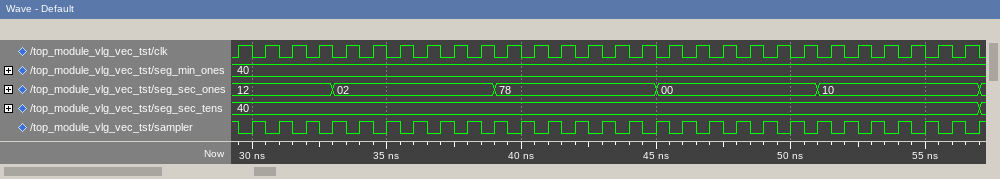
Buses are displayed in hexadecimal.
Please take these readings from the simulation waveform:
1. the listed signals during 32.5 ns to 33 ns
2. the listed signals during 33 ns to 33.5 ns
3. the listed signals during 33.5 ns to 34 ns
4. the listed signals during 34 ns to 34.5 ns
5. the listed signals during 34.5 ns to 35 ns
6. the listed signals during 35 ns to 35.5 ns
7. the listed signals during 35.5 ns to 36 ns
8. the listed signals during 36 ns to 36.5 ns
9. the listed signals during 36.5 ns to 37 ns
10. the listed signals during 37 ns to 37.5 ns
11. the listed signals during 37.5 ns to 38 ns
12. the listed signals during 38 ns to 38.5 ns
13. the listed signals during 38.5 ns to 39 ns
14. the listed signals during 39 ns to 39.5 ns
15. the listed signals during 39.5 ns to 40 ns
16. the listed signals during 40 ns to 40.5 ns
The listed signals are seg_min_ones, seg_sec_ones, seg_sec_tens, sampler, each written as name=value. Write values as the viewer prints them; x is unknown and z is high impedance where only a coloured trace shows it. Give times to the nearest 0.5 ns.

seg_min_ones=40, seg_sec_ones=12, seg_sec_tens=40, sampler=0
seg_min_ones=40, seg_sec_ones=02, seg_sec_tens=40, sampler=1
seg_min_ones=40, seg_sec_ones=02, seg_sec_tens=40, sampler=0
seg_min_ones=40, seg_sec_ones=02, seg_sec_tens=40, sampler=1
seg_min_ones=40, seg_sec_ones=02, seg_sec_tens=40, sampler=0
seg_min_ones=40, seg_sec_ones=02, seg_sec_tens=40, sampler=1
seg_min_ones=40, seg_sec_ones=02, seg_sec_tens=40, sampler=0
seg_min_ones=40, seg_sec_ones=02, seg_sec_tens=40, sampler=1
seg_min_ones=40, seg_sec_ones=02, seg_sec_tens=40, sampler=0
seg_min_ones=40, seg_sec_ones=02, seg_sec_tens=40, sampler=1
seg_min_ones=40, seg_sec_ones=02, seg_sec_tens=40, sampler=0
seg_min_ones=40, seg_sec_ones=02, seg_sec_tens=40, sampler=1
seg_min_ones=40, seg_sec_ones=02, seg_sec_tens=40, sampler=0
seg_min_ones=40, seg_sec_ones=78, seg_sec_tens=40, sampler=1
seg_min_ones=40, seg_sec_ones=78, seg_sec_tens=40, sampler=0
seg_min_ones=40, seg_sec_ones=78, seg_sec_tens=40, sampler=1
